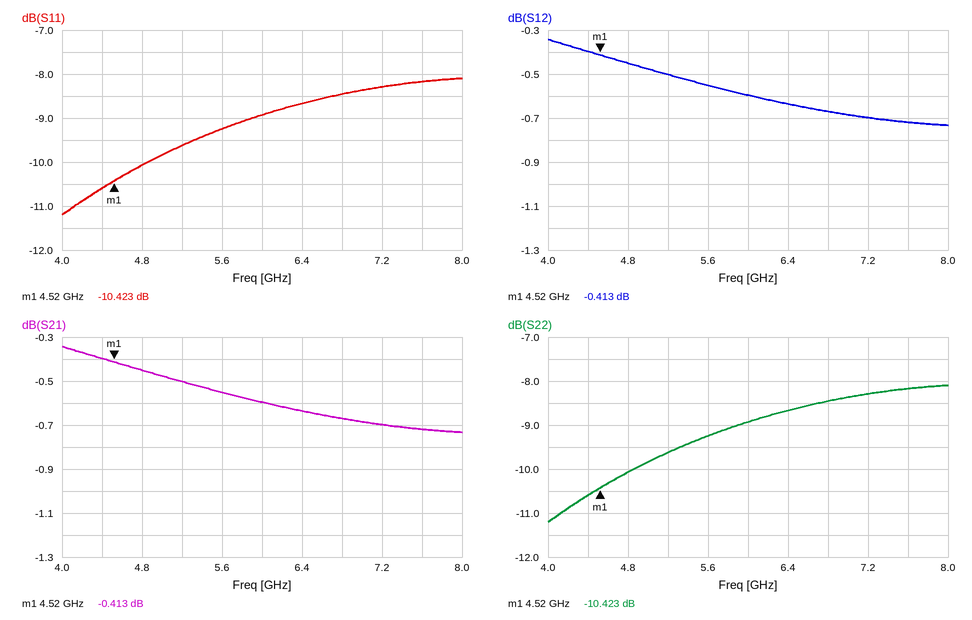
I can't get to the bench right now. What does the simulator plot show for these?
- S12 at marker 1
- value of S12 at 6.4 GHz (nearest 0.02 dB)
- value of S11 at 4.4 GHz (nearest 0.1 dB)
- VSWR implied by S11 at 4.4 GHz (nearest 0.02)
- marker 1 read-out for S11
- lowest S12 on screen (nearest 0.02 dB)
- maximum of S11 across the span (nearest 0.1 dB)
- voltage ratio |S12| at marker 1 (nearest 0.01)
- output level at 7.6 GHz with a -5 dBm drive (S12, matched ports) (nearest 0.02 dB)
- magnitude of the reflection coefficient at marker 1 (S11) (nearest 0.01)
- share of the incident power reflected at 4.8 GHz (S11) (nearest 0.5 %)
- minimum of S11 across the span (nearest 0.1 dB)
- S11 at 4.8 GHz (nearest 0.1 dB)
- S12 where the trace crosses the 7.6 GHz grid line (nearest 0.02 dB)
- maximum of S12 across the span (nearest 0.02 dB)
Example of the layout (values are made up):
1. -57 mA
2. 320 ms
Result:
1. -0.413 dB
2. -0.64 dB
3. -10.6 dB
4. 1.84
5. -10.423 dB
6. -0.74 dB
7. -8.1 dB
8. 0.95
9. -5.72 dBm
10. 0.30
11. 10.0 %
12. -11.2 dB
13. -10.1 dB
14. -0.72 dB
15. -0.34 dB
